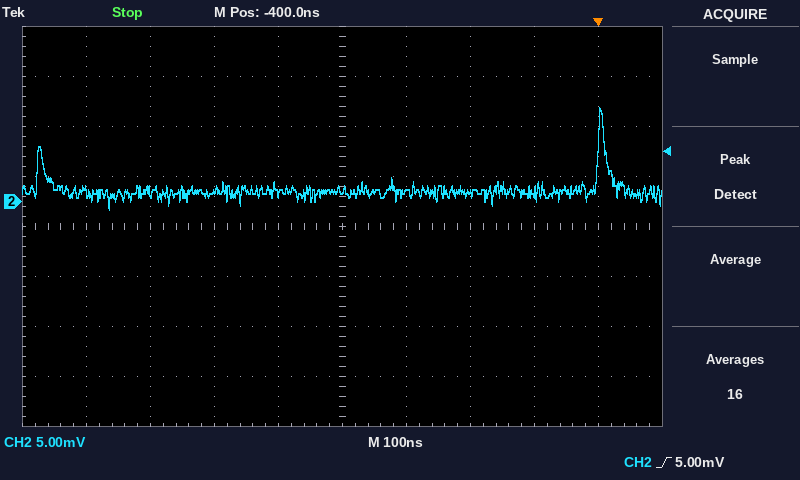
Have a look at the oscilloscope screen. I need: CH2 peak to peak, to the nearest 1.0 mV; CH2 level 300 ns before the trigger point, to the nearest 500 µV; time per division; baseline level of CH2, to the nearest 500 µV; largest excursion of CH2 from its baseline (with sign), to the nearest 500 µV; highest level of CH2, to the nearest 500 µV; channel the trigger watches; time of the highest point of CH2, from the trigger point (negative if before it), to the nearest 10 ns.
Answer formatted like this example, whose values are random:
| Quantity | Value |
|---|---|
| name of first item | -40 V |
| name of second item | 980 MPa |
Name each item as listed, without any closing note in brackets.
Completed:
| Quantity | Value |
|---|---|
| CH2 peak to peak, to the nearest 1.0 mV | 10.0 mV |
| CH2 level 300 ns before the trigger point, to the nearest 500 µV | 1.0 mV |
| time per division | 100 ns |
| baseline level of CH2, to the nearest 500 µV | 1.0 mV |
| largest excursion of CH2 from its baseline (with sign), to the nearest 500 µV | +8.5 mV |
| highest level of CH2, to the nearest 500 µV | 9.5 mV |
| channel the trigger watches | CH2 |
| time of the highest point of CH2, from the trigger point (negative if before it), to the nearest 10 ns | 0 ns |
